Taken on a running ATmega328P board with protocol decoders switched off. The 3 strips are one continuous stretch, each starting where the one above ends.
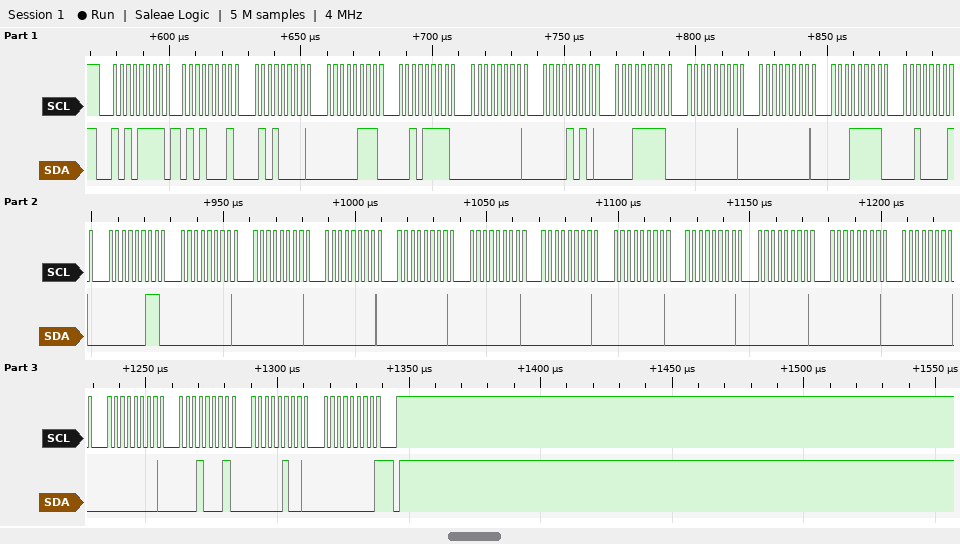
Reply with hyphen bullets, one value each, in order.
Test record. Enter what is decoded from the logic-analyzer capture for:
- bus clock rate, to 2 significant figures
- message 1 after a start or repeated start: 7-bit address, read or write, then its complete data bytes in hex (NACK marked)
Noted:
- 400 kHz
- 0x57 read: 51 50 07 2F 00 0A 1F 00 00 1F 21 03 00 00 00 00 00 00 00 00 00 00 00 00 11 04 00 NACK
